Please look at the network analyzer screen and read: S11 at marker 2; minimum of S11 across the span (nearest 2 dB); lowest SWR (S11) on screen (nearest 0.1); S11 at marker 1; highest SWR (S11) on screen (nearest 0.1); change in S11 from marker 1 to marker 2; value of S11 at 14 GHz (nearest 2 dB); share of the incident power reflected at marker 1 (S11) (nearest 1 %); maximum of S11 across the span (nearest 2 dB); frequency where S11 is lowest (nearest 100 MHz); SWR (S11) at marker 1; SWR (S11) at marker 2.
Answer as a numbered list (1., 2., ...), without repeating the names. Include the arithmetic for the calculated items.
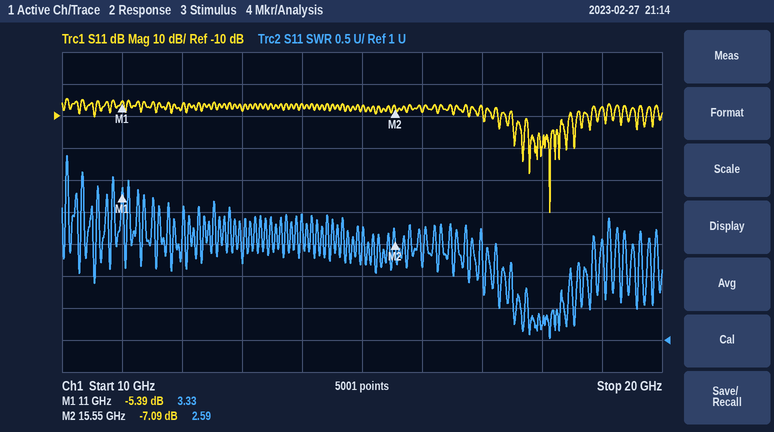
1. -7.09 dB
2. -40 dB
3. 1.0
4. -5.39 dB
5. 3.9
6. -7.09 − (-5.39) = -1.70 dB
7. -6 dB
8. 10^(-5.39/10) ≈ 29 %
9. -4 dB
10. 18.1 GHz
11. 3.33
12. 2.59
